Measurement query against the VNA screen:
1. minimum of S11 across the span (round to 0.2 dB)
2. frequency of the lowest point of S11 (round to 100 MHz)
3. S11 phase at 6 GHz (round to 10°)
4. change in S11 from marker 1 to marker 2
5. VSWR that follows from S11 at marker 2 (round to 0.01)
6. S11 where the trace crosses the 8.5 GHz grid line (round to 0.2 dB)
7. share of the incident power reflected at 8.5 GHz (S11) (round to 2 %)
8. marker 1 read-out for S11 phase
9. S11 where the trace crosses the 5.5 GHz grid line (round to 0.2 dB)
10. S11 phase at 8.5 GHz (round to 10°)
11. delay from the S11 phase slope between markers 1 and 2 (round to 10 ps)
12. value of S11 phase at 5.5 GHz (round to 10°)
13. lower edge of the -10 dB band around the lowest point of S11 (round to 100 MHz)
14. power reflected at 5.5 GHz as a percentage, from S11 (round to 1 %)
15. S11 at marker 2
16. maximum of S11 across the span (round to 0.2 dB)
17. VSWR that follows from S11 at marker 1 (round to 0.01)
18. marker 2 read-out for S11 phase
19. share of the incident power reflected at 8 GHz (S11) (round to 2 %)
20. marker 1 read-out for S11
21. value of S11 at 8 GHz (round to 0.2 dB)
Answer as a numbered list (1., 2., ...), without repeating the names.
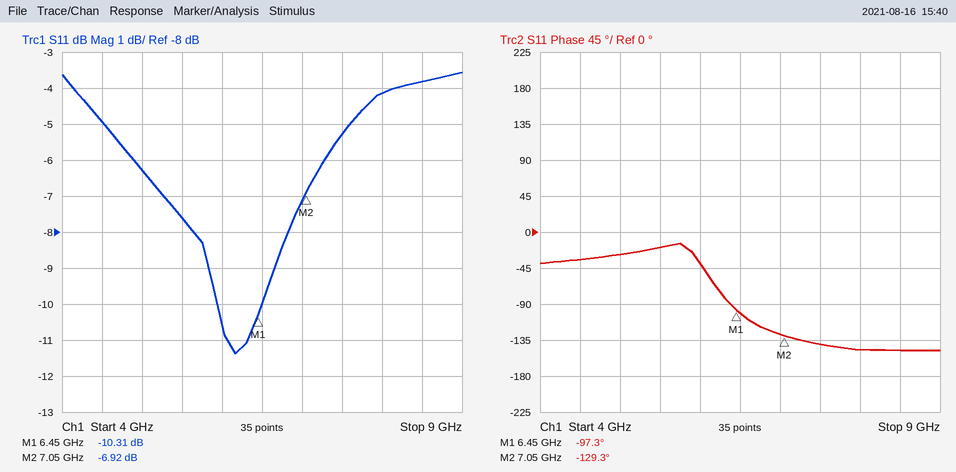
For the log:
1. -11.4 dB
2. 6.2 GHz
3. -40°
4. 3.39 dB
5. 2.64
6. -3.8 dB
7. 42 %
8. -97.3°
9. -7.6 dB
10. -150°
11. 150 ps
12. -20°
13. 5.9 GHz
14. 17 %
15. -6.92 dB
16. -3.6 dB
17. 1.88
18. -129.3°
19. 38 %
20. -10.31 dB
21. -4.2 dB
